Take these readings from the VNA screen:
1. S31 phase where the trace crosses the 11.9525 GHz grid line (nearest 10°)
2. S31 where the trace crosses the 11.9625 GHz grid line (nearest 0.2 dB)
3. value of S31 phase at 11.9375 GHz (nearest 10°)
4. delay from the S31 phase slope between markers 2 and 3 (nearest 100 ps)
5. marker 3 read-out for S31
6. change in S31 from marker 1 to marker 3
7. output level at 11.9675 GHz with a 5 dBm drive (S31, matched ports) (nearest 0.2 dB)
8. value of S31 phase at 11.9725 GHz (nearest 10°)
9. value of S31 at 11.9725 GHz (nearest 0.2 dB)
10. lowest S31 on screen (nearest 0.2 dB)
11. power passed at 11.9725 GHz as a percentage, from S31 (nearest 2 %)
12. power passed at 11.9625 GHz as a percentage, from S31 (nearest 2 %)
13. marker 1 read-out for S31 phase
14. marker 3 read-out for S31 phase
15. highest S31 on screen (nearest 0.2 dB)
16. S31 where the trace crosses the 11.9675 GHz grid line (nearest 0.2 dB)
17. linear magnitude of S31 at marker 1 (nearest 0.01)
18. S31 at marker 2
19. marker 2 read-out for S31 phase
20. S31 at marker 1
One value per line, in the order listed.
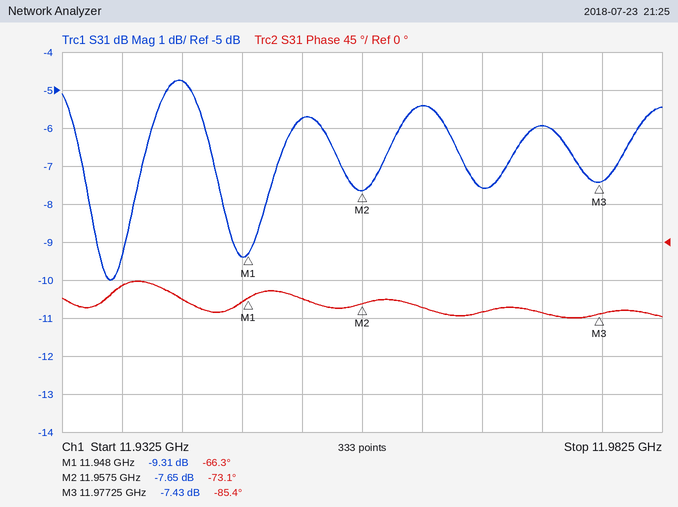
-70°
-5.4 dB
-50°
1.7 ns
-7.43 dB
1.88 dB
-2.6 dBm
-80°
-6.0 dB
-10.0 dB
26 %
28 %
-66.3°
-85.4°
-4.8 dB
-7.6 dB
0.34
-7.65 dB
-73.1°
-9.31 dB
